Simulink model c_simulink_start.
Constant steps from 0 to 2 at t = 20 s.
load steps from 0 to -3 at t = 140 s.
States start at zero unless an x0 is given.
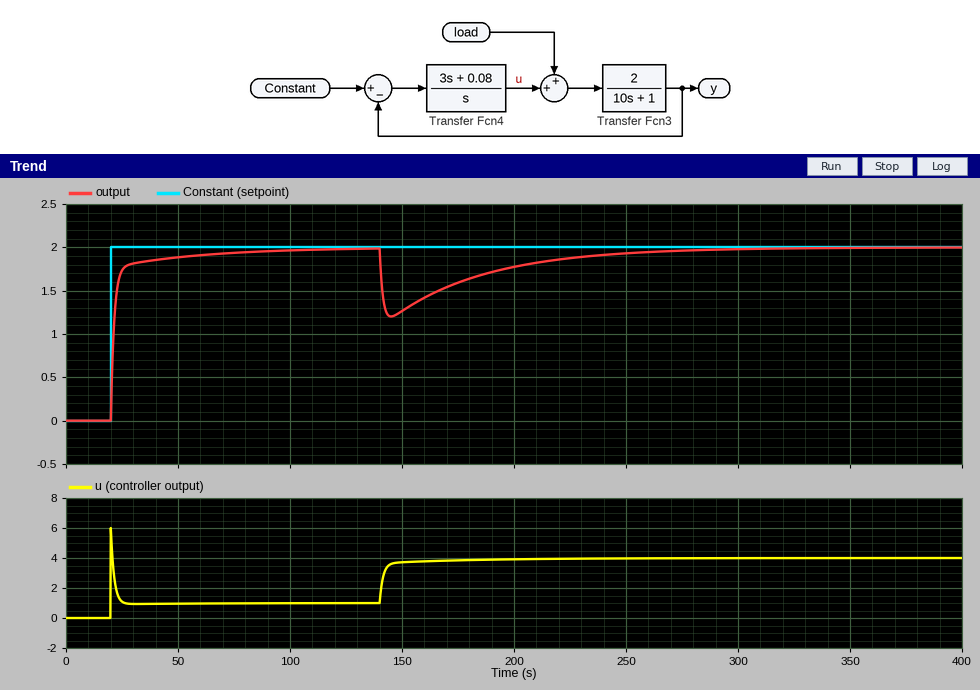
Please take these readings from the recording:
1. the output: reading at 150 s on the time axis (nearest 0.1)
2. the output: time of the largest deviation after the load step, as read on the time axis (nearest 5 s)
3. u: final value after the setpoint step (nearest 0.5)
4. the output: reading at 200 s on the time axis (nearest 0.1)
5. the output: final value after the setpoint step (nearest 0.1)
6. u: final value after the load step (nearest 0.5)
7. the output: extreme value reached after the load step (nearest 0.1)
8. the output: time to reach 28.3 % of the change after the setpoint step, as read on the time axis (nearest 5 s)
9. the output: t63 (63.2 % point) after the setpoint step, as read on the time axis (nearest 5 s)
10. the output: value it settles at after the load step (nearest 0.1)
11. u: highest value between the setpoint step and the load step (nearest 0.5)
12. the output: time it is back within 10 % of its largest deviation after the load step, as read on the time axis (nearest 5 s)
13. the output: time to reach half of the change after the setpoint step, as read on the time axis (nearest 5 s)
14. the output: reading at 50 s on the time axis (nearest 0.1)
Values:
1.3
145 s
1.0
1.8
2.0
4.0
1.2
20 s
20 s
2.0
6.0
245 s
20 s
1.9
